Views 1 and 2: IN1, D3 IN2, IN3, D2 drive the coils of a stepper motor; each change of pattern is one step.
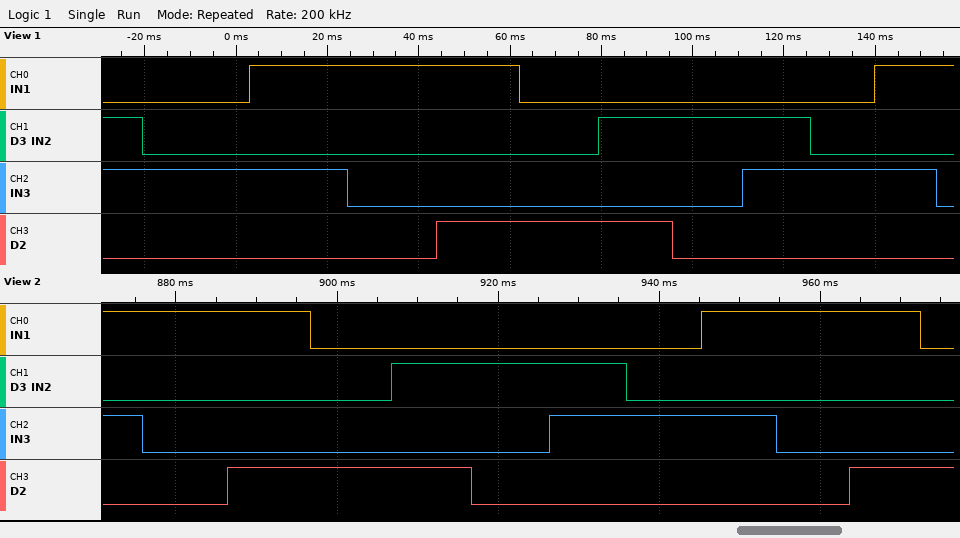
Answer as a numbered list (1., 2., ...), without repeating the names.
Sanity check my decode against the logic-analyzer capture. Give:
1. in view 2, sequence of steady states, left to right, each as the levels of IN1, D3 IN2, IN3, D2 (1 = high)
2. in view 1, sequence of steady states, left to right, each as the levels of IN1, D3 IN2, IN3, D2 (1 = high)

1. 1010 1000 1001 0001 0101 0100 0110 0010 1010 1000 1001 0001
2. 0110 0010 1010 1000 1001 0001 0101 0100 0110 0010 1010 1000
